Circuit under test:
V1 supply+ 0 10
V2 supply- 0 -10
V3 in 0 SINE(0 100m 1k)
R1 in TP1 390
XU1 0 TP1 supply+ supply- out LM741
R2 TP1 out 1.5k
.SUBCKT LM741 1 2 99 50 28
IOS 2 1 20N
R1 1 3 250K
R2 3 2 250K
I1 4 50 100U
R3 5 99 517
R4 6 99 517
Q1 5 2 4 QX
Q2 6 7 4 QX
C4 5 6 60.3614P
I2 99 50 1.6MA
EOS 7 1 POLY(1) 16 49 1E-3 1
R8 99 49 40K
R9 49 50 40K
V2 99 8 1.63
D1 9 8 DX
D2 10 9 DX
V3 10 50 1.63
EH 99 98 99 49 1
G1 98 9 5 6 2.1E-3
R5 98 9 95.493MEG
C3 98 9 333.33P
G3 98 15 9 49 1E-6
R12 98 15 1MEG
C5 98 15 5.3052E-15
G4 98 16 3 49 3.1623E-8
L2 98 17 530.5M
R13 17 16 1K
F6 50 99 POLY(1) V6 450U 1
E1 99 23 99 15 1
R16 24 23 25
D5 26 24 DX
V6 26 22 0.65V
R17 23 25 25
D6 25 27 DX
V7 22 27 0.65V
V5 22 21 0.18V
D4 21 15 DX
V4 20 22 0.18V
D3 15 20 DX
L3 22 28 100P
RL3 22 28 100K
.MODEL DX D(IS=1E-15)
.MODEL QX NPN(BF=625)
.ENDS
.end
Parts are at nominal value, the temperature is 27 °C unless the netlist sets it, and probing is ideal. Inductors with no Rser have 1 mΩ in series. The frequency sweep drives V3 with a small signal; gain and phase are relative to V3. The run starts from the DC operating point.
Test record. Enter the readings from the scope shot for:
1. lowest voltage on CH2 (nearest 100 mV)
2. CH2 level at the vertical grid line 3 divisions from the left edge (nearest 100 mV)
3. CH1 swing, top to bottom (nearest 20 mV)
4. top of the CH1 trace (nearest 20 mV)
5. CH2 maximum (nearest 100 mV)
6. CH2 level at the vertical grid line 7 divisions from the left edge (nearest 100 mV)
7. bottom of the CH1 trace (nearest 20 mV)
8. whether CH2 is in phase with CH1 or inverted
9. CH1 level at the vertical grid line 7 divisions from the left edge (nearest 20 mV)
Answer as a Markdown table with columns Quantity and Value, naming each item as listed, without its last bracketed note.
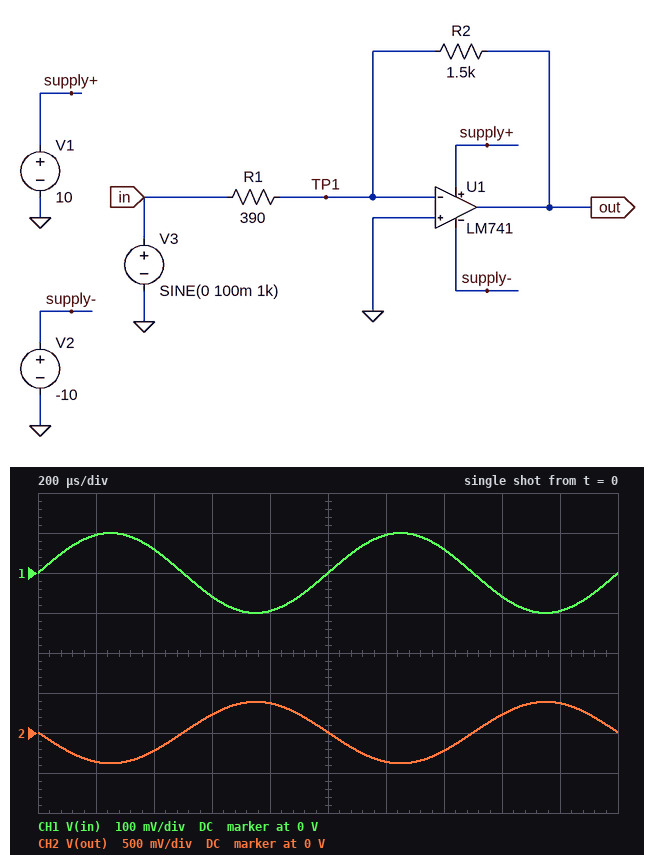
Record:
| Quantity | Value |
|---|---|
| lowest voltage on CH2 | -400 mV |
| CH2 level at the vertical grid line 3 divisions from the left edge | 200 mV |
| CH1 swing, top to bottom | 200 mV |
| top of the CH1 trace | 100 mV |
| CH2 maximum | 400 mV |
| CH2 level at the vertical grid line 7 divisions from the left edge | -200 mV |
| bottom of the CH1 trace | -100 mV |
| whether CH2 is in phase with CH1 or inverted | inverted |
| CH1 level at the vertical grid line 7 divisions from the left edge | 60 mV |
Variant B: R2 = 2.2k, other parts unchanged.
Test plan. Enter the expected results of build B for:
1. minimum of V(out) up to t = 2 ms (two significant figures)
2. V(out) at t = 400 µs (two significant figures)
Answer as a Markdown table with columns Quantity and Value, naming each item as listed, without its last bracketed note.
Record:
| Quantity | Value |
|---|---|
| minimum of V(out) up to t = 2 ms | -560 mV |
| V(out) at t = 400 µs | -330 mV |
